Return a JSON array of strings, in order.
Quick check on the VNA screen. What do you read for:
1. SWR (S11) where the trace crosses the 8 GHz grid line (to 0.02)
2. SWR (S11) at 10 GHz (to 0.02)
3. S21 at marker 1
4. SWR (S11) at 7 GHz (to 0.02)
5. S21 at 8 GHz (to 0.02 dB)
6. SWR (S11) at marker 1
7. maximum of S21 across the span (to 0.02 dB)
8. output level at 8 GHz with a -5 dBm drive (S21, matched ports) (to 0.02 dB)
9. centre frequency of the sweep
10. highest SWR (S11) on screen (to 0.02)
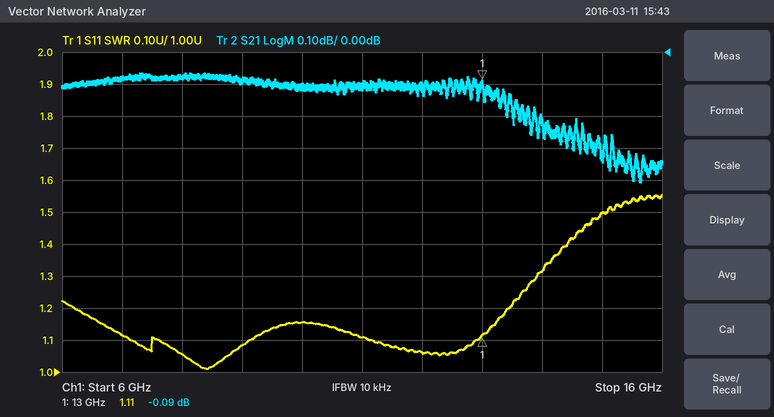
["1.06", "1.16", "-0.09 dB", "1.12", "-0.08 dB", "1.11", "-0.06 dB", "-5.08 dBm", "11 GHz", "1.56"]
